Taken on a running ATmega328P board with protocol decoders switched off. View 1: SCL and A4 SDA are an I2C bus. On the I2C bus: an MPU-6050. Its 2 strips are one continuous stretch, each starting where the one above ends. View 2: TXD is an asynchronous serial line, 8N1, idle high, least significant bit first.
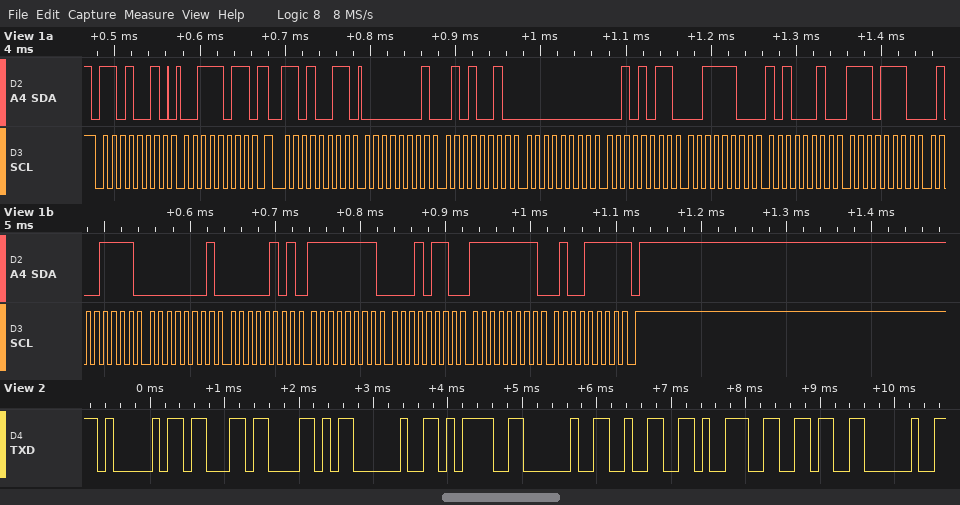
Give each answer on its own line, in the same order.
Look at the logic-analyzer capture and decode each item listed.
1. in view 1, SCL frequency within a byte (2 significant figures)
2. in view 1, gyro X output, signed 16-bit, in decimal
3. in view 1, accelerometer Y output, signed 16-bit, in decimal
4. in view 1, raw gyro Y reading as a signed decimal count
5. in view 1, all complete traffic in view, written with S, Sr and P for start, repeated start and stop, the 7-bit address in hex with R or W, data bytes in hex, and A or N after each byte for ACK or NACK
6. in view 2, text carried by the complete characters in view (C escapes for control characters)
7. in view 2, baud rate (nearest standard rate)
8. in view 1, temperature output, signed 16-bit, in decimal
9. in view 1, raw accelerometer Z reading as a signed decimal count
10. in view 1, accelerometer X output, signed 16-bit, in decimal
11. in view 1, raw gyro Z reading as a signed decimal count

100 kHz
261
43
-234
S 69W A 3B A Sr 69R A 01 A 52 A 00 A 2B A 3C A A2 A EE A 4F A 01 A 05 A FF A 16 A FF A 4F N P
"AcX = 296 "
9600 baud
-4529
15522
338
-177
